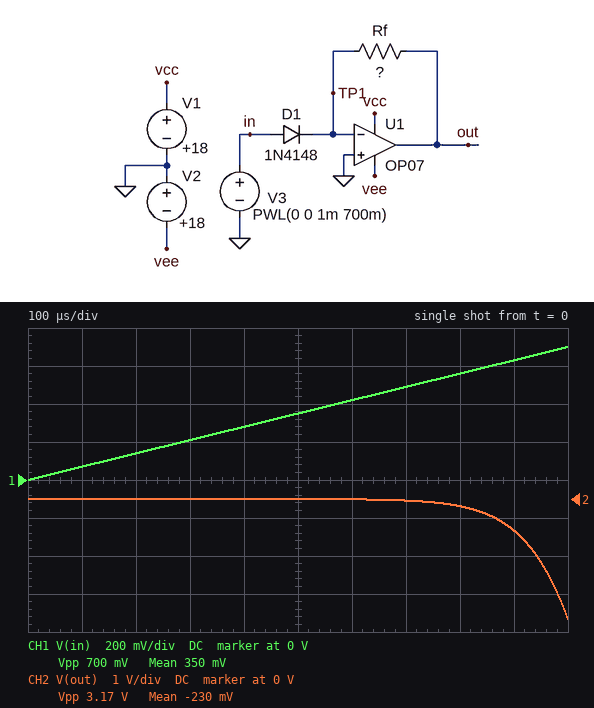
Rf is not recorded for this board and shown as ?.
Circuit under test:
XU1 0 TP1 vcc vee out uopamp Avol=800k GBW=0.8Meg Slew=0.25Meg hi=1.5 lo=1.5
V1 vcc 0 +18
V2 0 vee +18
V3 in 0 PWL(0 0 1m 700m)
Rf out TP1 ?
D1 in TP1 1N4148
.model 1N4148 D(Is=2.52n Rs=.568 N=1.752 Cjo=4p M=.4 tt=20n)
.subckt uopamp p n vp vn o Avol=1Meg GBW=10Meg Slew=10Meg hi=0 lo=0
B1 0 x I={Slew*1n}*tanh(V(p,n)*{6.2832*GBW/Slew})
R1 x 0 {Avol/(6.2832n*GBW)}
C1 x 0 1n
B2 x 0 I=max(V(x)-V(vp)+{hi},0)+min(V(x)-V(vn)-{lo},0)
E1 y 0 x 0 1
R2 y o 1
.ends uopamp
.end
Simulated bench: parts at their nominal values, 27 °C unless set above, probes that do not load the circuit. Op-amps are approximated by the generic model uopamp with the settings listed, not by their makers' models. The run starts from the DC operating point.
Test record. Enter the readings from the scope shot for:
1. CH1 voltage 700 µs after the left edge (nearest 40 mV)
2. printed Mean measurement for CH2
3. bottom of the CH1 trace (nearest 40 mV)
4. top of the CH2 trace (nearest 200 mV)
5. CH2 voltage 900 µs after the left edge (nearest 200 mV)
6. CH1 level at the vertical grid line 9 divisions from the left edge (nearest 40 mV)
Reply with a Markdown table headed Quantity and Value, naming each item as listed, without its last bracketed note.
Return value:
| Quantity | Value |
|---|---|
| CH1 voltage 700 µs after the left edge | 480 mV |
| printed Mean measurement for CH2 | -230 mV |
| bottom of the CH1 trace | 0 V |
| top of the CH2 trace | 0 V |
| CH2 voltage 900 µs after the left edge | -800 mV |
| CH1 level at the vertical grid line 9 divisions from the left edge | 640 mV |
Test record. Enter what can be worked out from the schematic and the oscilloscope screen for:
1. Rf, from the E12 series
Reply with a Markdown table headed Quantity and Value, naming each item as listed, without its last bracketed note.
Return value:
| Quantity | Value |
|---|---|
| Rf, from the E12 series | 330 Ω |
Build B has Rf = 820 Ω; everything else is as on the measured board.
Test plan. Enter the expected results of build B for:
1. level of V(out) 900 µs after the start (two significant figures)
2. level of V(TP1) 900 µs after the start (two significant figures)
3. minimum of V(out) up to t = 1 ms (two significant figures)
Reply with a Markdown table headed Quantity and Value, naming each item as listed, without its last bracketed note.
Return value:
| Quantity | Value |
|---|---|
| level of V(out) 900 µs after the start | -1.9 V |
| level of V(TP1) 900 µs after the start | 5.3 mV |
| minimum of V(out) up to t = 1 ms | -6.8 V |
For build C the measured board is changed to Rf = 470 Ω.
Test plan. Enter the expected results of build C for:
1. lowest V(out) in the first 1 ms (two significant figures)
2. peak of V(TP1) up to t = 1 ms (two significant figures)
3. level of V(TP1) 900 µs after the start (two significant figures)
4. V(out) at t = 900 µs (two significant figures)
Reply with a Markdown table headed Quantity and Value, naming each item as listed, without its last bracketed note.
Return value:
| Quantity | Value |
|---|---|
| lowest V(out) in the first 1 ms | -4.3 V |
| peak of V(TP1) up to t = 1 ms | 10 mV |
| level of V(TP1) 900 µs after the start | 3.3 mV |
| V(out) at t = 900 µs | -1.2 V |
